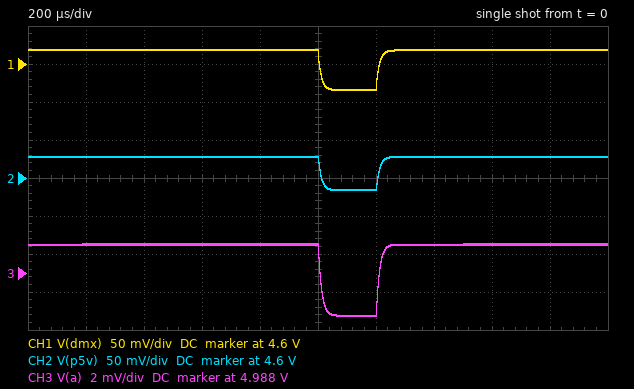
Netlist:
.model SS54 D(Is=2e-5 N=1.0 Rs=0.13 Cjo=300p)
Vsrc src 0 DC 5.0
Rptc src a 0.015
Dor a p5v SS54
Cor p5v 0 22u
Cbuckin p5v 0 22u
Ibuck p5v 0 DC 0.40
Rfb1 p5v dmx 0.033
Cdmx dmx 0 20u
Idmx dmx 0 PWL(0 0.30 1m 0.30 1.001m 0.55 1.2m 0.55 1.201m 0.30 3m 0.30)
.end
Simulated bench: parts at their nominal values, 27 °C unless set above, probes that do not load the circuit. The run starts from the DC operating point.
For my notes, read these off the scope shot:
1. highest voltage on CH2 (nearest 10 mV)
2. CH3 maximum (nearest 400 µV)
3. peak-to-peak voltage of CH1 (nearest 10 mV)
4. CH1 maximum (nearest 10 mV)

4.63 V
4.9896 V
50 mV
4.62 V
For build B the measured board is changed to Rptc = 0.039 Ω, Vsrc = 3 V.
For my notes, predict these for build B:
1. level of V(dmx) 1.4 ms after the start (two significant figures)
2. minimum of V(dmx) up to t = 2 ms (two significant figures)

2.6 V
2.5 V
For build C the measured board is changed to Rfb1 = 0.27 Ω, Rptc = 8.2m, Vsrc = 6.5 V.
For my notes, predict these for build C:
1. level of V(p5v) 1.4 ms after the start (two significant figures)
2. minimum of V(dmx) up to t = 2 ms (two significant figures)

6.1 V
5.9 V
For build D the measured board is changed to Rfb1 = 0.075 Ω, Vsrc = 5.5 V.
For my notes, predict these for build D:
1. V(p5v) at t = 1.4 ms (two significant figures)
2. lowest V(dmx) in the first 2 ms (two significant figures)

5.1 V
5.0 V
